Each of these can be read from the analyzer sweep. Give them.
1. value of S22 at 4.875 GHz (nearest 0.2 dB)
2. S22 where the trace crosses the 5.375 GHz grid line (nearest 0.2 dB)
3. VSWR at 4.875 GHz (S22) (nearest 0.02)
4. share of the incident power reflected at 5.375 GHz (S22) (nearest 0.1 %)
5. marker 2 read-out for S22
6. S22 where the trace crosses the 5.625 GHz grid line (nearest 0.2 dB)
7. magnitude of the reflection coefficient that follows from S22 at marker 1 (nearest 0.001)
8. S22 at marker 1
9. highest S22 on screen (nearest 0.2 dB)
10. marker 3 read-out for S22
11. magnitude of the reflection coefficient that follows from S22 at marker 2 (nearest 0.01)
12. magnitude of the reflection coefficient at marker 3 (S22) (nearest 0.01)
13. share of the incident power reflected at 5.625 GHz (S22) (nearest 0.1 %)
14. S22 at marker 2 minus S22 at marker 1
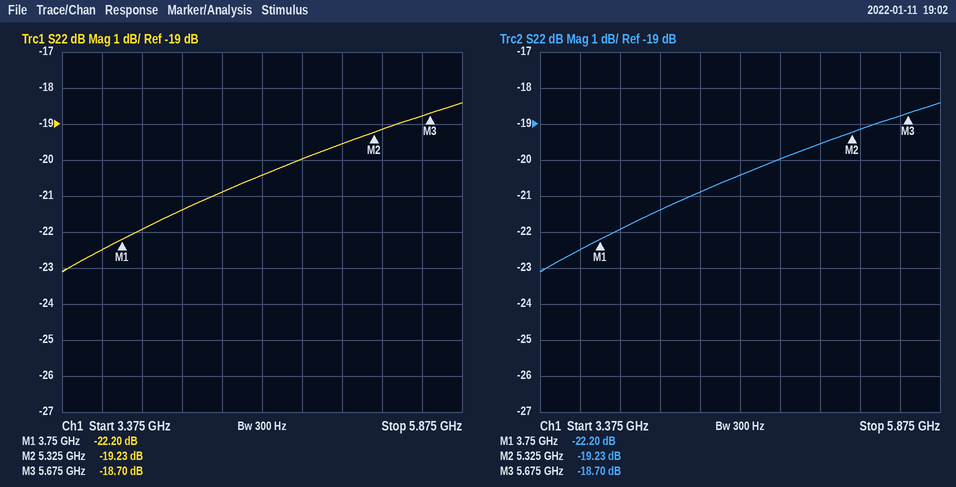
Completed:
-20.0 dB
-19.2 dB
1.22
1.2 %
-19.23 dB
-18.8 dB
0.078
-22.20 dB
-18.4 dB
-18.70 dB
0.11
0.12
1.3 %
2.97 dB
